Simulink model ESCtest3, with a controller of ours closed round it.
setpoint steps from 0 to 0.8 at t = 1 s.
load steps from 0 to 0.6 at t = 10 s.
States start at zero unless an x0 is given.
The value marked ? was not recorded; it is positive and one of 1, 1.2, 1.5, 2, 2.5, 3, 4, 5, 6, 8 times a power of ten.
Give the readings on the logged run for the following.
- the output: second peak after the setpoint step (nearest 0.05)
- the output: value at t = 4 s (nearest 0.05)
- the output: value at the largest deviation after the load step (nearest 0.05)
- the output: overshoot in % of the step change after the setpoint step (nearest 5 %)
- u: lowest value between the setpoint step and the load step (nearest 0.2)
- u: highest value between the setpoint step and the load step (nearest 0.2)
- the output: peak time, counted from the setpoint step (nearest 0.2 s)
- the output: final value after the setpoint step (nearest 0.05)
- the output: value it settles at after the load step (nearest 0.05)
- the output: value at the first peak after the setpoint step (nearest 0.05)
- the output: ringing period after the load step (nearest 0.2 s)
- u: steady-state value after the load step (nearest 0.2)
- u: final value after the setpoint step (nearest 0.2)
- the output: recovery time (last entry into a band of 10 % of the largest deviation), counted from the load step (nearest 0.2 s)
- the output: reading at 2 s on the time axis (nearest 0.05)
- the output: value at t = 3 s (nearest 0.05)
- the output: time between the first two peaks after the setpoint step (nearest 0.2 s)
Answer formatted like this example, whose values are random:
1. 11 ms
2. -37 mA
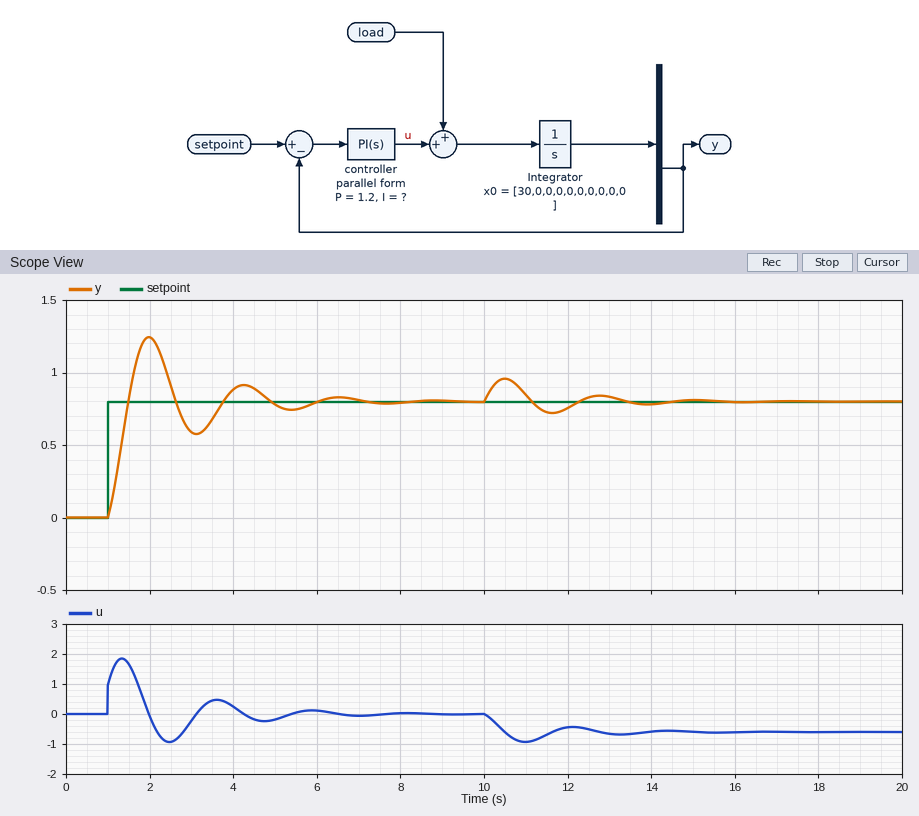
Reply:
1. 0.90
2. 0.90
3. 0.95
4. 55 %
5. -1.0
6. 1.8
7. 1.0 s
8. 0.80
9. 0.80
10. 1.25
11. 2.2 s
12. -0.6
13. 0.0
14. 4.2 s
15. 1.25
16. 0.60
17. 2.2 s
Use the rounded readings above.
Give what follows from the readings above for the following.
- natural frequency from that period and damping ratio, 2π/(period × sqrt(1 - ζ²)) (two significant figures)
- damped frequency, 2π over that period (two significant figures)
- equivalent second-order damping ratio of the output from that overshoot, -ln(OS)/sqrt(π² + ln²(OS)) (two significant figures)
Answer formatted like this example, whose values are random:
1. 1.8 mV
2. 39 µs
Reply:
1. 2.9 rad/s
2. 2.9 rad/s
3. 0.19
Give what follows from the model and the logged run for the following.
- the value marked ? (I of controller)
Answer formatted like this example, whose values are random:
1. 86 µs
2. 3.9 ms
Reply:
1. 8
